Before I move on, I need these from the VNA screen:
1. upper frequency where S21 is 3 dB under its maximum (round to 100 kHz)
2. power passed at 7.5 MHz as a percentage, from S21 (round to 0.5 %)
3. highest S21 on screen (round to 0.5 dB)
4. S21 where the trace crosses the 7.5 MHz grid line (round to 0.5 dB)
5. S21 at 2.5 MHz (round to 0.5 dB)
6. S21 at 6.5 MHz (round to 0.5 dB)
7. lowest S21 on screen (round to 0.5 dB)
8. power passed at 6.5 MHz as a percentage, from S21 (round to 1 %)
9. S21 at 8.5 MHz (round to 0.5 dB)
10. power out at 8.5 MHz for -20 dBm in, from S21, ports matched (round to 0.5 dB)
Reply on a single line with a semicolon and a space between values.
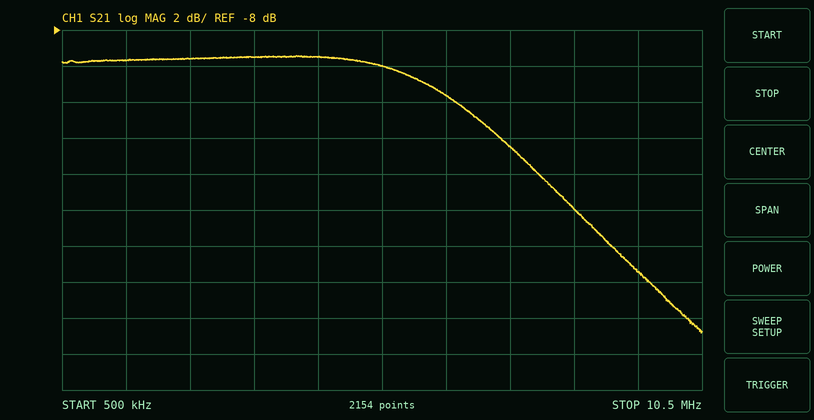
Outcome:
6.8 MHz; 3.5 %; -9.5 dB; -14.5 dB; -9.5 dB; -11.5 dB; -25.0 dB; 7 %; -18.0 dB; -38.0 dBm
